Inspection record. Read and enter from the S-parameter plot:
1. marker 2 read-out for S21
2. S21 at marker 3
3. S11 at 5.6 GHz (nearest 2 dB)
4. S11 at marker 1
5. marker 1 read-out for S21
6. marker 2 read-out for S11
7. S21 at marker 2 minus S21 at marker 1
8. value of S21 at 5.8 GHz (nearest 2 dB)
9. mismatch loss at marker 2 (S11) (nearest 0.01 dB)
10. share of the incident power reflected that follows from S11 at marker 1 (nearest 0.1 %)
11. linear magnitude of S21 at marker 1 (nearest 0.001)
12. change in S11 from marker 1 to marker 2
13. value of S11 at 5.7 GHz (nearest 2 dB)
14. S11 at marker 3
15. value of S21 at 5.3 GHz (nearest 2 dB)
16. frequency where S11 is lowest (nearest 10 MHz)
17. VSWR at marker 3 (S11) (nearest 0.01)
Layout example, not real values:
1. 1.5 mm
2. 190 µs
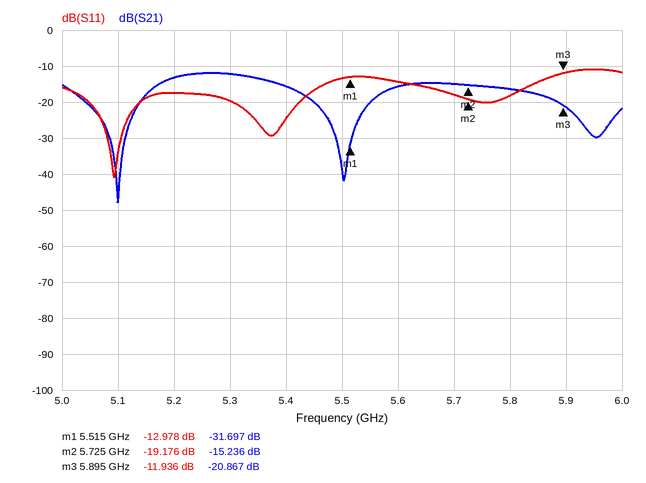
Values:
1. -15.236 dB
2. -20.867 dB
3. -14 dB
4. -12.978 dB
5. -31.697 dB
6. -19.176 dB
7. 16.461 dB
8. -16 dB
9. 0.05 dB
10. 5.0 %
11. 0.026
12. -6.198 dB
13. -18 dB
14. -11.936 dB
15. -12 dB
16. 5.09 GHz
17. 1.68
